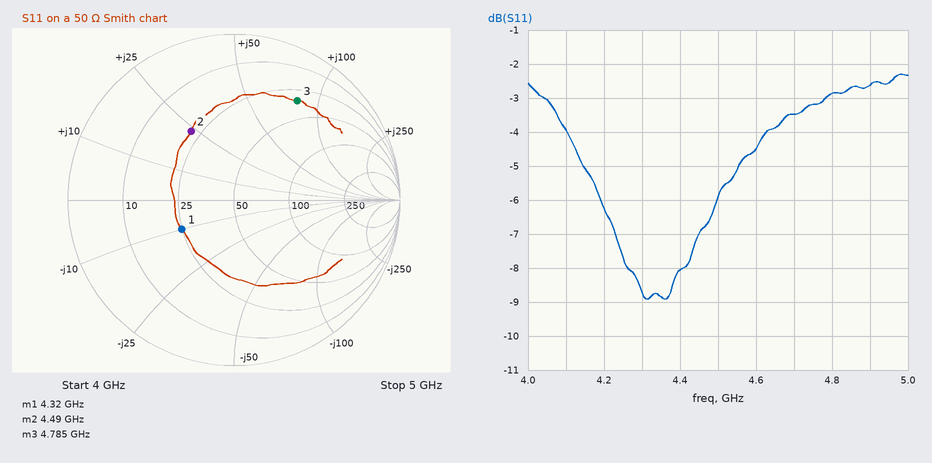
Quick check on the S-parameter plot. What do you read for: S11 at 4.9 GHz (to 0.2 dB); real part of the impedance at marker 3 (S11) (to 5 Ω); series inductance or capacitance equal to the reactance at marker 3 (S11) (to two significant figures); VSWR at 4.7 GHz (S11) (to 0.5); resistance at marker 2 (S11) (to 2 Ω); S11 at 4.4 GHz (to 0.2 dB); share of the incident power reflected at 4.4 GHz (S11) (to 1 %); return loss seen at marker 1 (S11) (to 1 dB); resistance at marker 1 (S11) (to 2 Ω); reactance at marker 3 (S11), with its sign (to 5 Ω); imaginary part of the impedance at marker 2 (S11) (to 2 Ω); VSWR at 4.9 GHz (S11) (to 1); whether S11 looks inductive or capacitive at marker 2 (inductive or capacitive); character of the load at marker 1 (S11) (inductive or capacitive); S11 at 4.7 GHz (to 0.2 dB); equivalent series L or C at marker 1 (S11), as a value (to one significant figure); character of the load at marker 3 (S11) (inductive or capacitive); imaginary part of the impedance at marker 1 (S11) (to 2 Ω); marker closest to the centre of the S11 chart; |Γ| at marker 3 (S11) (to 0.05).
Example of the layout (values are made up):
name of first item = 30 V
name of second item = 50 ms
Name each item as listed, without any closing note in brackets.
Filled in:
S11 at 4.9 GHz = -2.6 dB
real part of the impedance at marker 3 (S11) = 35 Ω
series inductance or capacitance equal to the reactance at marker 3 (S11) = 2.7 nH
VSWR at 4.7 GHz (S11) = 5.0
resistance at marker 2 (S11) = 22 Ω
S11 at 4.4 GHz = -8.0 dB
share of the incident power reflected at 4.4 GHz (S11) = 16 %
return loss seen at marker 1 (S11) = 9 dB
resistance at marker 1 (S11) = 24 Ω
reactance at marker 3 (S11), with its sign = +80 Ω
imaginary part of the impedance at marker 2 (S11) = +24 Ω
VSWR at 4.9 GHz (S11) = 7
whether S11 looks inductive or capacitive at marker 2 = inductive
character of the load at marker 1 (S11) = capacitive
S11 at 4.7 GHz = -3.4 dB
equivalent series L or C at marker 1 (S11), as a value = 4 pF
character of the load at marker 3 (S11) = inductive
imaginary part of the impedance at marker 1 (S11) = -10 Ω
marker closest to the centre of the S11 chart = marker 1
|Γ| at marker 3 (S11) = 0.70
